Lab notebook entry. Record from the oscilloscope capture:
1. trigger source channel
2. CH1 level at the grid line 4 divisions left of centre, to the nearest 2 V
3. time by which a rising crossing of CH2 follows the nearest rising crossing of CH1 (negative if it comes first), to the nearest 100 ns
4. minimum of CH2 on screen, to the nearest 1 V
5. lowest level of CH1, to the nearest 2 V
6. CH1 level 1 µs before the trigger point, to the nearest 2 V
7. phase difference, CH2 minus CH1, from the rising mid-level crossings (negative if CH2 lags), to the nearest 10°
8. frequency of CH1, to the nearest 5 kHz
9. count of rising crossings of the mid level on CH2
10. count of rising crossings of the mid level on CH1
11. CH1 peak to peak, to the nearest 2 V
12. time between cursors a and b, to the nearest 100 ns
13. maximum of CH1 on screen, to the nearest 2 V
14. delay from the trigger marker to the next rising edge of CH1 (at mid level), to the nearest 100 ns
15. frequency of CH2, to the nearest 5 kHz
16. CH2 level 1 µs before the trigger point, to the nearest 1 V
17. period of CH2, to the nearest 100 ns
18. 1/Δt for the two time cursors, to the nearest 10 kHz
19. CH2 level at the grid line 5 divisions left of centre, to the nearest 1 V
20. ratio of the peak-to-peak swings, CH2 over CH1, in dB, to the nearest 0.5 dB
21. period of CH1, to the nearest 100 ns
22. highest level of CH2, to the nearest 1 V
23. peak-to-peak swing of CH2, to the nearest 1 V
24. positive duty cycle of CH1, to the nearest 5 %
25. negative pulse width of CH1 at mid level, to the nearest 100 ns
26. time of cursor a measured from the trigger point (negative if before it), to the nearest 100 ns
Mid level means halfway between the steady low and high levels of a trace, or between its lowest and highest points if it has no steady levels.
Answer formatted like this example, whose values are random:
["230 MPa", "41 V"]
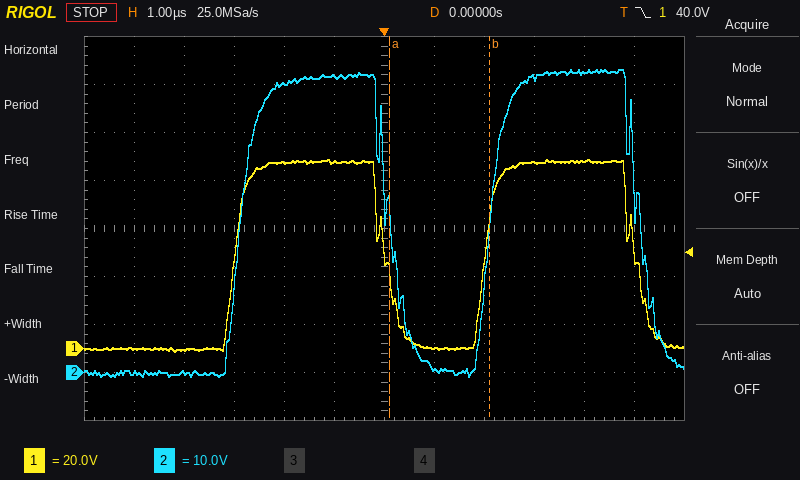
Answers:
["CH1", "0 V", "+100 ns", "-1 V", "-2 V", "78 V", "-10°", "200 kHz", "2", "2", "80 V", "2.0 µs", "78 V", "2.0 µs", "200 kHz", "62 V", "5.0 µs", "500 kHz", "0 V", "-2.0 dB", "5.0 µs", "63 V", "64 V", "60 %", "2.0 µs", "+100 ns"]
